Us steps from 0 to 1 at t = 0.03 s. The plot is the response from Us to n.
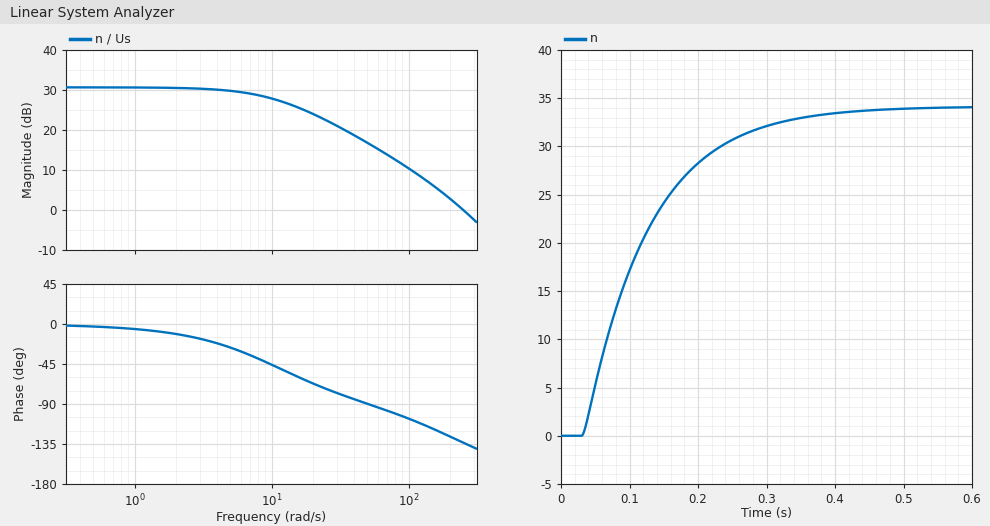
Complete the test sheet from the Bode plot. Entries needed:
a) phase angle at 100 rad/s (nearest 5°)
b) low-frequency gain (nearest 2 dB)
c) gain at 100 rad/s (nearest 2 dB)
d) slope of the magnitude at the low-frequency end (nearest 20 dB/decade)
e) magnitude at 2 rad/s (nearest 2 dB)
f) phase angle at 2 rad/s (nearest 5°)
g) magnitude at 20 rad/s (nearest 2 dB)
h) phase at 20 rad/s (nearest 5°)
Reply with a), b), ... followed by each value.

a) -105°
b) 30 dB
c) 10 dB
d) 0 dB/decade
e) 30 dB
f) -10°
g) 24 dB
h) -65°
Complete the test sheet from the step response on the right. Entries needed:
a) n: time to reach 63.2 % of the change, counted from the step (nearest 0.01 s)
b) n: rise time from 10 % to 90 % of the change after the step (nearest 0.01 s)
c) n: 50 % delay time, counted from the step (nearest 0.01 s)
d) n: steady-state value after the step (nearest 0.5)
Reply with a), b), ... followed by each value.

a) 0.10 s
b) 0.21 s
c) 0.07 s
d) 34.0
